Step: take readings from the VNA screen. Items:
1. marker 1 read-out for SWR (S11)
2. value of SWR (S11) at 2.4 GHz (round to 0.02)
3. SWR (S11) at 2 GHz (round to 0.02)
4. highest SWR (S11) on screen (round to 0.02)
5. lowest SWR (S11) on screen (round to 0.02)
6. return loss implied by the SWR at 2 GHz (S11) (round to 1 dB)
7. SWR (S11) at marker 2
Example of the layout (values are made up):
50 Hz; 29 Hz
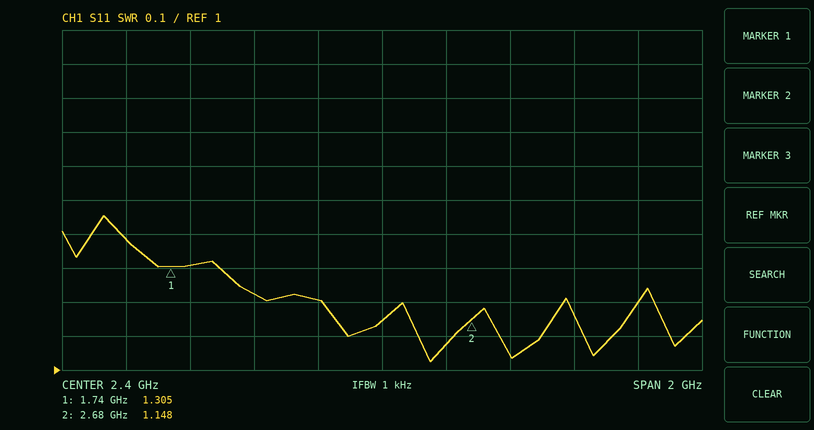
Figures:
1.305; 1.14; 1.22; 1.46; 1.02; 20 dB; 1.148
